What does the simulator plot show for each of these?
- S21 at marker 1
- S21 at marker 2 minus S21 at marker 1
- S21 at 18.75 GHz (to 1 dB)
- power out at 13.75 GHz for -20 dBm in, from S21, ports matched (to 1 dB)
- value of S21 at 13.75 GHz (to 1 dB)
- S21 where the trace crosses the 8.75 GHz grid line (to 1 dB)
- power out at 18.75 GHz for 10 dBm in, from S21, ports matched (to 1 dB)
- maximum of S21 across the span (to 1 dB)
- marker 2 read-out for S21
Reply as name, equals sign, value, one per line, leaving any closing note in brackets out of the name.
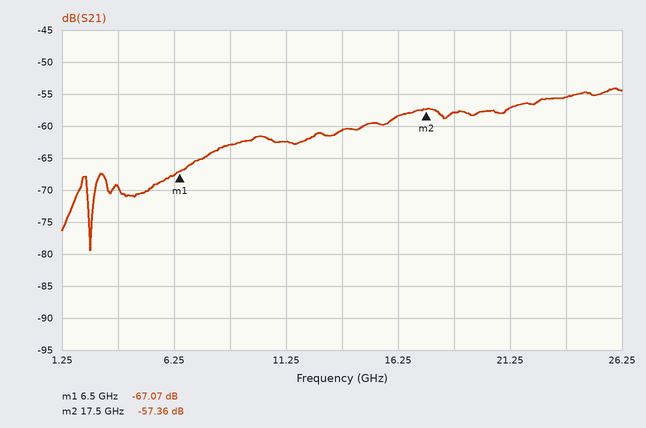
S21 at marker 1 = -67.07 dB
S21 at marker 2 minus S21 at marker 1 = 9.71 dB
S21 at 18.75 GHz = -58 dB
power out at 13.75 GHz for -20 dBm in, from S21, ports matched = -81 dBm
value of S21 at 13.75 GHz = -61 dB
S21 where the trace crosses the 8.75 GHz grid line = -63 dB
power out at 18.75 GHz for 10 dBm in, from S21, ports matched = -48 dBm
maximum of S21 across the span = -54 dB
marker 2 read-out for S21 = -57.36 dB
